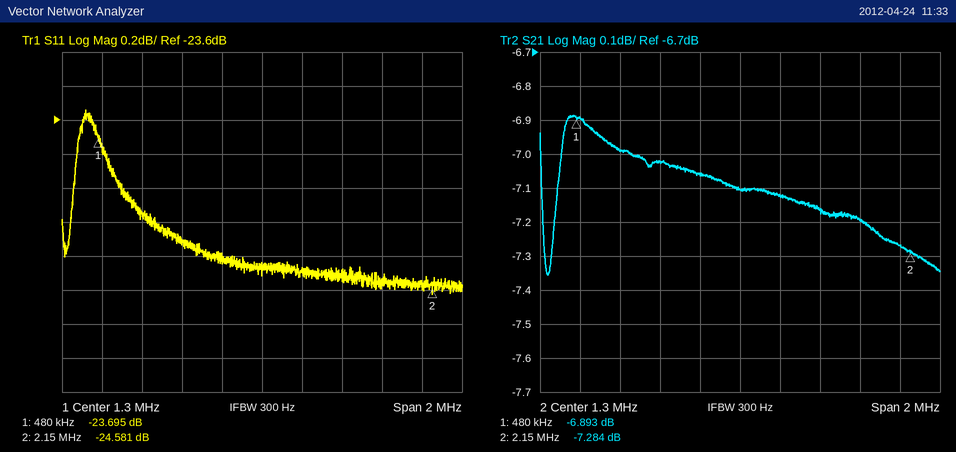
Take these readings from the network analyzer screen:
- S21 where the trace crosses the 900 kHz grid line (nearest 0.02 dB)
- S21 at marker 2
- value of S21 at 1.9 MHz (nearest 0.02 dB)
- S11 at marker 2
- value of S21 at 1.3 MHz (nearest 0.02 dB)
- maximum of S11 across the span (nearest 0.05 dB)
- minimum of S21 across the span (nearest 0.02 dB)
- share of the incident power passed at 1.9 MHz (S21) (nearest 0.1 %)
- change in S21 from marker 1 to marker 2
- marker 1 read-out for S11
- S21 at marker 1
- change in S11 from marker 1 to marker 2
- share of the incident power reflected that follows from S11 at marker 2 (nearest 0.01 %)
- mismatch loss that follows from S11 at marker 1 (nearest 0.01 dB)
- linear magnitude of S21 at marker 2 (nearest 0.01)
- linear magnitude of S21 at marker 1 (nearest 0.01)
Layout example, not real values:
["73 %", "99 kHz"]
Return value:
["-7.02 dB", "-7.284 dB", "-7.20 dB", "-24.581 dB", "-7.10 dB", "-23.55 dB", "-7.36 dB", "19.1 %", "-0.391 dB", "-23.695 dB", "-6.893 dB", "-0.886 dB", "0.35 %", "0.02 dB", "0.43", "0.45"]
